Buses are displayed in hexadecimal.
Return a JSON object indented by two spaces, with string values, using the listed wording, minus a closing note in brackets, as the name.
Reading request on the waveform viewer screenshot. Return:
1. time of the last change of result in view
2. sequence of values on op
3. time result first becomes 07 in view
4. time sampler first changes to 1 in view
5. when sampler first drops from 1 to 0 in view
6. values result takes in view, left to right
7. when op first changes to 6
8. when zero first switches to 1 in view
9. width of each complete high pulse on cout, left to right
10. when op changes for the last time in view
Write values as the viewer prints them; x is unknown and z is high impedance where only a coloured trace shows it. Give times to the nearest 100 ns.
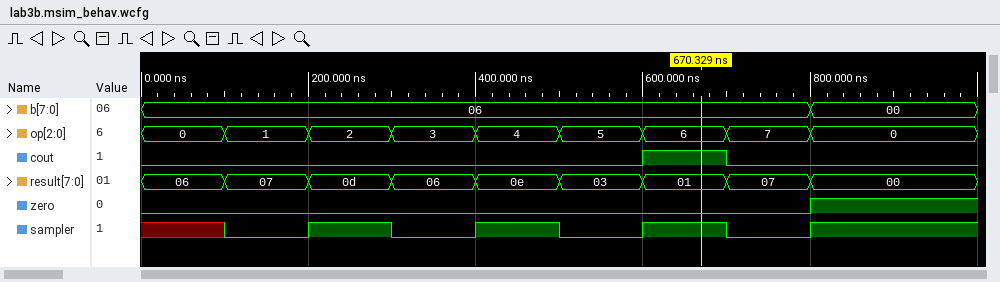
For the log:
{
  "time of the last change of result in view": "800 ns",
  "sequence of values on op": "0, 1, 2, 3, 4, 5, 6, 7, 0",
  "time result first becomes 07 in view": "100 ns",
  "time sampler first changes to 1 in view": "200 ns",
  "when sampler first drops from 1 to 0 in view": "300 ns",
  "values result takes in view, left to right": "06, 07, 0d, 06, 0e, 03, 01, 07, 00",
  "when op first changes to 6": "600 ns",
  "when zero first switches to 1 in view": "800 ns",
  "width of each complete high pulse on cout, left to right": "100 ns",
  "when op changes for the last time in view": "800 ns"
}
